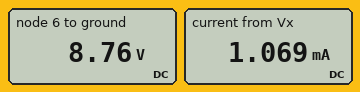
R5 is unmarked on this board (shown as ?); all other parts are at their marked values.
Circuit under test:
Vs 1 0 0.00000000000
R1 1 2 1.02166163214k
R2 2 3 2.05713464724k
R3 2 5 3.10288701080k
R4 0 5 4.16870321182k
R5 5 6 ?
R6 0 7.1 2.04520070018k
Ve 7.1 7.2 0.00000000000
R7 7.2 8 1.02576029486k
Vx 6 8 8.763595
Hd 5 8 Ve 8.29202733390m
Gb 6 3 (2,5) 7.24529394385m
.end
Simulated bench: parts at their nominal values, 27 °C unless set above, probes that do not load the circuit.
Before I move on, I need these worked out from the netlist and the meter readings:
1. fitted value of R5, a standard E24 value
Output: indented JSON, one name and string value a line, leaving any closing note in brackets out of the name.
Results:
{
  "fitted value of R5, a standard E24 value": "8.2 kΩ"
}
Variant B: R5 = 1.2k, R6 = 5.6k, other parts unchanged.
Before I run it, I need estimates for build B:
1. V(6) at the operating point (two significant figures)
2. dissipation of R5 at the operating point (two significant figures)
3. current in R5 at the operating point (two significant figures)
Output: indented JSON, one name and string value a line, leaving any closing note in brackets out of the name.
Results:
{
  "V(6) at the operating point": "8.8 V",
  "dissipation of R5 at the operating point": "64 mW",
  "current in R5 at the operating point": "7.3 mA"
}
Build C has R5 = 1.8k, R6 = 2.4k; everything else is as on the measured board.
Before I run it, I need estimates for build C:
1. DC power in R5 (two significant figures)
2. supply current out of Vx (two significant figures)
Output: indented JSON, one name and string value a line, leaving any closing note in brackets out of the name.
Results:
{
  "DC power in R5": "43 mW",
  "supply current out of Vx": "4.9 mA"
}
